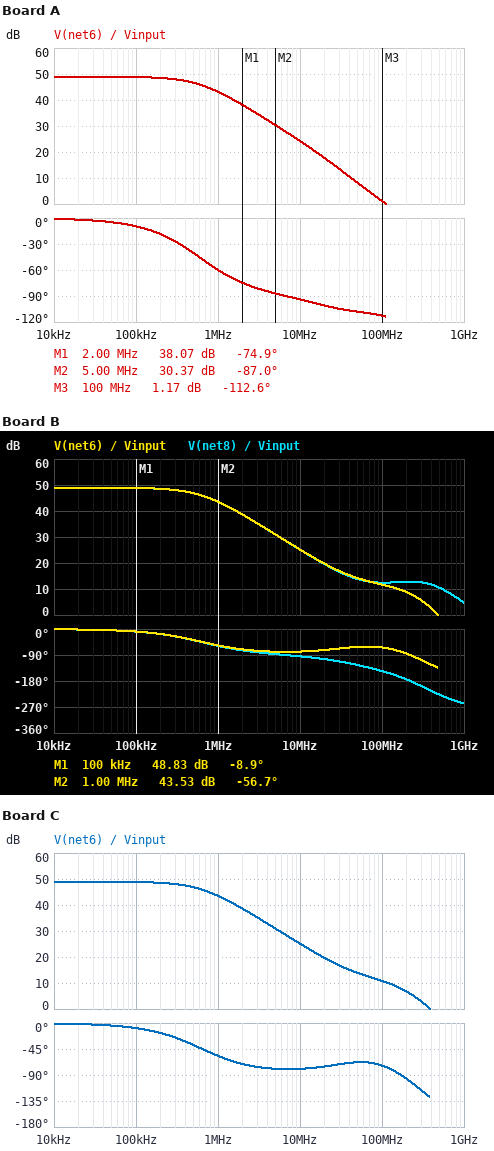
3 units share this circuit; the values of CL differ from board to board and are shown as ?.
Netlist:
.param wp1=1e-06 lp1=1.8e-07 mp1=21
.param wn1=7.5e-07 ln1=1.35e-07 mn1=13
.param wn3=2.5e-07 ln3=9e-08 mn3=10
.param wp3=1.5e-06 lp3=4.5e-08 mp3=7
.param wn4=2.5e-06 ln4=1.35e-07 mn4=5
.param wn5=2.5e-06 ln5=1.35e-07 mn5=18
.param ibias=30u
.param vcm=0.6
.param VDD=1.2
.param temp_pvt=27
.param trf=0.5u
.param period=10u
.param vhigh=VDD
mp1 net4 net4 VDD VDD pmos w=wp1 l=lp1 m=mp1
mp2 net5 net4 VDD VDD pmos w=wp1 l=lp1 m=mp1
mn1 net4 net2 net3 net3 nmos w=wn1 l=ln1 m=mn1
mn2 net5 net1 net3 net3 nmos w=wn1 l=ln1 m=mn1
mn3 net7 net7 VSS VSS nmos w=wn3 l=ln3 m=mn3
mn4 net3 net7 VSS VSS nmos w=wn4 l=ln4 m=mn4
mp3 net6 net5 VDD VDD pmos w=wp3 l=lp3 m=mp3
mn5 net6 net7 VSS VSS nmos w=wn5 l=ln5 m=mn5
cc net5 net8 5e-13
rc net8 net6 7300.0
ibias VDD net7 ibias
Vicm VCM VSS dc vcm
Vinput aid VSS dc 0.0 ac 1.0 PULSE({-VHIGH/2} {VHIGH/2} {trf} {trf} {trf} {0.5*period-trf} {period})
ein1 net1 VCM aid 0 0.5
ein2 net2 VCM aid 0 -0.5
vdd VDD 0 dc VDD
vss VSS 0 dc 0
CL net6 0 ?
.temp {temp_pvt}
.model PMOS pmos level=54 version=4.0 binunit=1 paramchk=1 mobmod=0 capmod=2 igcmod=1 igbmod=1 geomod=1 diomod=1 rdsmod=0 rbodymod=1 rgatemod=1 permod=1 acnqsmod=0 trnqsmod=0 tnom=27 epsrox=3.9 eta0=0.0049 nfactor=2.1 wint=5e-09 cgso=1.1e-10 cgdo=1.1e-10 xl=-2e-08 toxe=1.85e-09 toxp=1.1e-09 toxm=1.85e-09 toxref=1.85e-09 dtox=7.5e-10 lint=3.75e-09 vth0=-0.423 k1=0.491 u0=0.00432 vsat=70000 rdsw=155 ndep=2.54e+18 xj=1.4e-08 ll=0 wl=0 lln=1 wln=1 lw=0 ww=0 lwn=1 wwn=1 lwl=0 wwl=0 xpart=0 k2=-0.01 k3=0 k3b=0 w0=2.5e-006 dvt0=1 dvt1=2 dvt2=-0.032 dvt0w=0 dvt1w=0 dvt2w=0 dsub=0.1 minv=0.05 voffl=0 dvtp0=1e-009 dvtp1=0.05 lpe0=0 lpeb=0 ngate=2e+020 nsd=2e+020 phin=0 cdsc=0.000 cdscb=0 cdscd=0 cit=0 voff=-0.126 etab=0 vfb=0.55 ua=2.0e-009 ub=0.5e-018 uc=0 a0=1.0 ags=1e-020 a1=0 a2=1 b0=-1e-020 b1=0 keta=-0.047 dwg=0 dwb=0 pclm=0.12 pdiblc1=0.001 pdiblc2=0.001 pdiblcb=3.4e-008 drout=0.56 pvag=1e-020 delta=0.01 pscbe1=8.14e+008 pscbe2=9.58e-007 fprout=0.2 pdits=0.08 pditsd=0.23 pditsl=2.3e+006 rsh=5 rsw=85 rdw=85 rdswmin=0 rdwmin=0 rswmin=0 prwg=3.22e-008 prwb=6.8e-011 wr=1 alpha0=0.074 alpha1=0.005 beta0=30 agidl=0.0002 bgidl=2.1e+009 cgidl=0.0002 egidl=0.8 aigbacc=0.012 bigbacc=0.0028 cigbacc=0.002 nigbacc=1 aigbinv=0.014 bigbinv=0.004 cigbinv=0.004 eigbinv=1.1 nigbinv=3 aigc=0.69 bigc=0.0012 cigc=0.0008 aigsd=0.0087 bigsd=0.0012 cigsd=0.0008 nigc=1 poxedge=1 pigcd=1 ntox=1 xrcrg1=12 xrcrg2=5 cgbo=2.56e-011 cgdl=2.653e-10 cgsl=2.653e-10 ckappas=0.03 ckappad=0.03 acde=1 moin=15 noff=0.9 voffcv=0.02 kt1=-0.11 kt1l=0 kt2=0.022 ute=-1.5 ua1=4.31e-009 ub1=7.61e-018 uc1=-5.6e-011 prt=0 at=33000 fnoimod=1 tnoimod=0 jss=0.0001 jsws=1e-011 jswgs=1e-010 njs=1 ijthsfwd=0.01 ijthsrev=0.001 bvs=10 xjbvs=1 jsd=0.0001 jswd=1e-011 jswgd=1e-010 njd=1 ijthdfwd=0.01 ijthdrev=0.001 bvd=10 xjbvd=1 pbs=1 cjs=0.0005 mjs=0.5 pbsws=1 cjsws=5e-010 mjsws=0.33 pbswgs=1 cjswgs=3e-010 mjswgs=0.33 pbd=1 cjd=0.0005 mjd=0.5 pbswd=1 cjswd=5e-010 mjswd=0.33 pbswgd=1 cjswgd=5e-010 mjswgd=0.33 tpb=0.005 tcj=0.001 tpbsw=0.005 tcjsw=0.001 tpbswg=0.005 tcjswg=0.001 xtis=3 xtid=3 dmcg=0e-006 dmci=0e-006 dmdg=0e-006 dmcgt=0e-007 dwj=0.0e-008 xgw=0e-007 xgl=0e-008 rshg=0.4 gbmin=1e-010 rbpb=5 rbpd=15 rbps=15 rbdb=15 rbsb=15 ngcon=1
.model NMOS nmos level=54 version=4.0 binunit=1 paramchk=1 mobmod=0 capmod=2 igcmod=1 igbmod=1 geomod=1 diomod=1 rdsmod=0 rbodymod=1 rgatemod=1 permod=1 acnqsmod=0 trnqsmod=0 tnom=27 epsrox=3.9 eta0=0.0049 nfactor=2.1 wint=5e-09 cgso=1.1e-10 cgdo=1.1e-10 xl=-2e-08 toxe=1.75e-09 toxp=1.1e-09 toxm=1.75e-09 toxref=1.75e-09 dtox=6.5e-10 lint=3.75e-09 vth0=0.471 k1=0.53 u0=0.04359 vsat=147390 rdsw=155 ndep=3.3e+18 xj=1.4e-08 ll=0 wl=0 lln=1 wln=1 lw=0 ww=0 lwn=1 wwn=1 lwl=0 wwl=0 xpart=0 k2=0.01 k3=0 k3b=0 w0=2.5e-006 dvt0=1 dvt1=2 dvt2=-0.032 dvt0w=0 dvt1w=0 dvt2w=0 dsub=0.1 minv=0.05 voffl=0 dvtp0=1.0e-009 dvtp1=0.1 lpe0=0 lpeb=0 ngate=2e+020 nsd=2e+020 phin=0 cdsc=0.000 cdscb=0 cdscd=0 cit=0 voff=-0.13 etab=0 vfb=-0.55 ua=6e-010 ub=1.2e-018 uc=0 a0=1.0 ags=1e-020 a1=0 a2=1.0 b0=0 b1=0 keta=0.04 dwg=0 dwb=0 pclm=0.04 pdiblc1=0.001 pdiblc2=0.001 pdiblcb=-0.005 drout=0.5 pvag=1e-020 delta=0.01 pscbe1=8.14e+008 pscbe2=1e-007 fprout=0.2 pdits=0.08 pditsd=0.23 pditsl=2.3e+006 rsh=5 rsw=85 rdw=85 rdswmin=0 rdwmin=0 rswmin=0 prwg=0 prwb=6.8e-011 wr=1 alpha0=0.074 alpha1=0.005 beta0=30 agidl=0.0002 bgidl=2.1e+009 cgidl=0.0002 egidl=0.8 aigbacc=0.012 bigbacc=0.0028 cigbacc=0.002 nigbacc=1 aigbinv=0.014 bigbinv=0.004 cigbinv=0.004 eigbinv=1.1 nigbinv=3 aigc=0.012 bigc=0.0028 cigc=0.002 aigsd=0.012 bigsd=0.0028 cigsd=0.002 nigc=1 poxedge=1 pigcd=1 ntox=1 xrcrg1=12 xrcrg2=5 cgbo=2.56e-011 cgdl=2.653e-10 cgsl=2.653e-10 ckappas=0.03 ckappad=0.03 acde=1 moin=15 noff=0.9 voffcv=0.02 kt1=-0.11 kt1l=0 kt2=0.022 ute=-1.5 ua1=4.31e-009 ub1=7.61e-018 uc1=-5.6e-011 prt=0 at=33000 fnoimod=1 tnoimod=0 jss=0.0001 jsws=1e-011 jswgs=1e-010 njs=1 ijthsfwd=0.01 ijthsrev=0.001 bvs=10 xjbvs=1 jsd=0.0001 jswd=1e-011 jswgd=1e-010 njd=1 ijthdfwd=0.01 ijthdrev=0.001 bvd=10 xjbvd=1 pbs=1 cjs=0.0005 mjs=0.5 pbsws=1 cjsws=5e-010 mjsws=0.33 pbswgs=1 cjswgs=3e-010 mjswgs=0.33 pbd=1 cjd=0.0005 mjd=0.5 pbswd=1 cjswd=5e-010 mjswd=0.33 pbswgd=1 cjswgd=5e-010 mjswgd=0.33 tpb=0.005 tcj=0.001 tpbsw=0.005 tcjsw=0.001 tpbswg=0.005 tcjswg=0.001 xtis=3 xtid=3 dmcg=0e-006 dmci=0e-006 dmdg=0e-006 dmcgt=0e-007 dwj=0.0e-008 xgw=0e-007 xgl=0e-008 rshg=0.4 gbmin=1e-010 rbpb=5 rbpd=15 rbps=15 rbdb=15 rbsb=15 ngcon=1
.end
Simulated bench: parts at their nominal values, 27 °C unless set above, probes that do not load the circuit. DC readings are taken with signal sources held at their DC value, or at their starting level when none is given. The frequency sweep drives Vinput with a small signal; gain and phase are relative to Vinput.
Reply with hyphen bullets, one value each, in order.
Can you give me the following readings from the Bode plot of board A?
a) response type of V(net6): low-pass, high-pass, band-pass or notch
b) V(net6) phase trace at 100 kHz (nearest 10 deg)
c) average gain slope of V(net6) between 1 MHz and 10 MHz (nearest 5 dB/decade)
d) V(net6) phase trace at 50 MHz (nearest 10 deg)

- low-pass
- -10 deg
- -20 dB/decade
- -110 deg
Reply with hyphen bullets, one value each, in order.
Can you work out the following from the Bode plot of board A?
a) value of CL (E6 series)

- 22 pF
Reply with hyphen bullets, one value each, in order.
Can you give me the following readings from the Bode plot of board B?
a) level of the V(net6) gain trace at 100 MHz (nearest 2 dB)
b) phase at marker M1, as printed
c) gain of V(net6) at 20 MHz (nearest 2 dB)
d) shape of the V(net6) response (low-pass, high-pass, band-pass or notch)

- 12 dB
- -8.9 deg
- 20 dB
- low-pass
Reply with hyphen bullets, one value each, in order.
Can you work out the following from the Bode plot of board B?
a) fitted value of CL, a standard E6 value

- 3.3 pF
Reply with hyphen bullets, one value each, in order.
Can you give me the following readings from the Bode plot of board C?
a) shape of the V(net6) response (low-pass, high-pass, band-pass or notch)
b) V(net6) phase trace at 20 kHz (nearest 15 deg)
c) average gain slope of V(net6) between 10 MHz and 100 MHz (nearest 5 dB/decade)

- low-pass
- 0 deg
- -15 dB/decade
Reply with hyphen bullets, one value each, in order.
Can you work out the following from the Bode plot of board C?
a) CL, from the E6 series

- 4.7 pF
